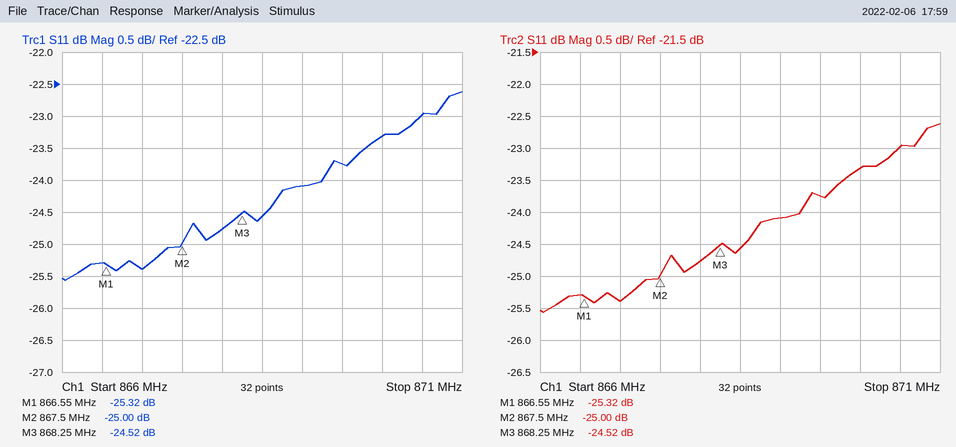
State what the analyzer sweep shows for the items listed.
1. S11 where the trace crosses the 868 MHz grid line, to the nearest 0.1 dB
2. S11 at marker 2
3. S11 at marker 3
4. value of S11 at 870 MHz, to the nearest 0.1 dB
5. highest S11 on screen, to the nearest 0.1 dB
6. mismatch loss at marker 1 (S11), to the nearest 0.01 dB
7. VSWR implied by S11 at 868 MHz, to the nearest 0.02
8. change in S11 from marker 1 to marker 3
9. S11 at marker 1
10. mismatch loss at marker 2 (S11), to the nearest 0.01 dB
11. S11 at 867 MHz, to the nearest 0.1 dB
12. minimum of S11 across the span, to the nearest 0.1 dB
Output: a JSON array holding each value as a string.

["-24.8 dB", "-25.00 dB", "-24.52 dB", "-23.3 dB", "-22.6 dB", "0.01 dB", "1.12", "0.80 dB", "-25.32 dB", "0.01 dB", "-25.4 dB", "-25.6 dB"]
